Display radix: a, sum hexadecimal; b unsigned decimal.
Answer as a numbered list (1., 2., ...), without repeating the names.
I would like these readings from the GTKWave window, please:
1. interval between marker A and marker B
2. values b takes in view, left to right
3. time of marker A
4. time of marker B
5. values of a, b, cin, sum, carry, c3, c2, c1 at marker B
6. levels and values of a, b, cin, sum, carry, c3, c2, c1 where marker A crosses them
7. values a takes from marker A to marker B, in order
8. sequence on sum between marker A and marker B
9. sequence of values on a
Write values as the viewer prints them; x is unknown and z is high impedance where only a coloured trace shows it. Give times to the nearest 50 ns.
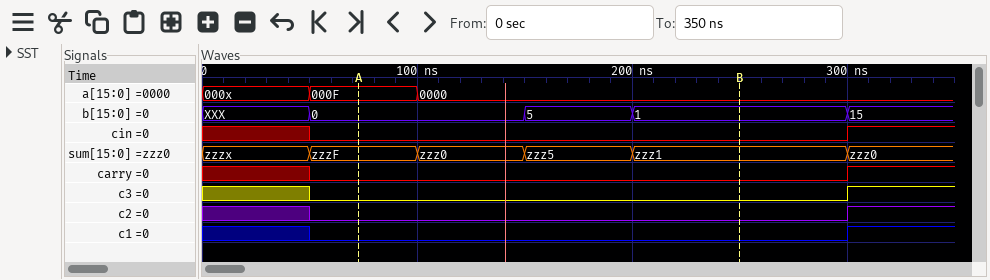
1. 200 ns
2. XXX, 0, 5, 1, 15
3. 50 ns
4. 250 ns
5. a=0000, b=1, cin=0, sum=zzz1, carry=0, c3=0, c2=0, c1=0
6. a=000F, b=0, cin=0, sum=zzzF, carry=0, c3=0, c2=0, c1=0
7. 000F, 0000
8. zzzF, zzz0, zzz5, zzz1
9. 000x, 000F, 0000
